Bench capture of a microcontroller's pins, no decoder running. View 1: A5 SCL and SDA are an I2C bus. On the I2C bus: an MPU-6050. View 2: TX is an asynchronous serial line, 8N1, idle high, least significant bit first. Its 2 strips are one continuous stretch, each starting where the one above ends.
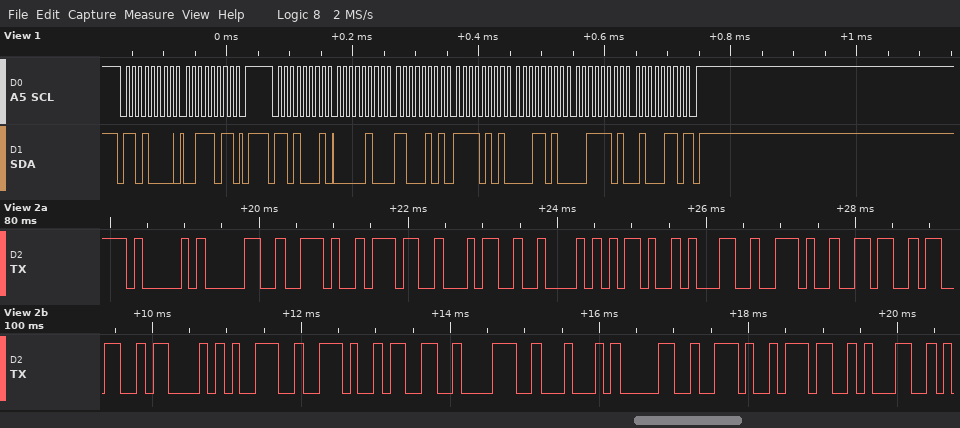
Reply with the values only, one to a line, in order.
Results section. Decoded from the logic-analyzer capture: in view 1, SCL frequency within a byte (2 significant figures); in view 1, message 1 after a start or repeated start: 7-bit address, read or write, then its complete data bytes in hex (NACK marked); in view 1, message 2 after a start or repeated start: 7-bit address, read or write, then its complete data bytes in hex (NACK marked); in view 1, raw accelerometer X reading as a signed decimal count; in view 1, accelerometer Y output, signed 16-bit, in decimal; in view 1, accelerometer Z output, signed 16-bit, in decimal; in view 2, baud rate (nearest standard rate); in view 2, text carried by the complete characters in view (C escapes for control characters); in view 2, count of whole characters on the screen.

100 kHz
0x68 write: 3B
0x68 read: 04 C5 F5 1A 3D 46 NACK
1221
-2790
15686
9600 baud
"A0.74B-1.63C9.38D0.71"
21
